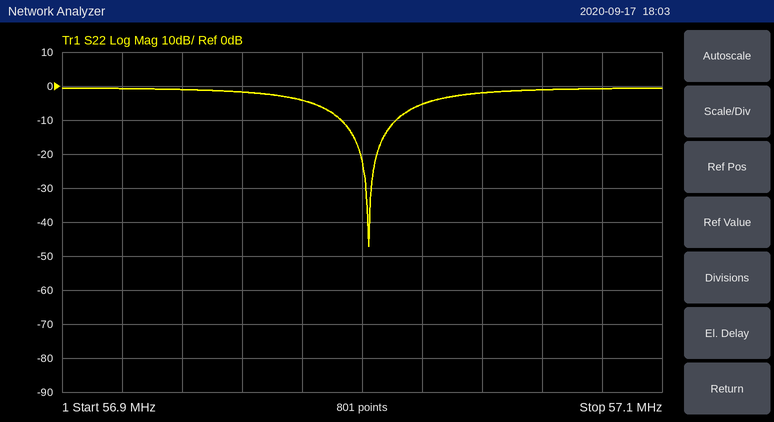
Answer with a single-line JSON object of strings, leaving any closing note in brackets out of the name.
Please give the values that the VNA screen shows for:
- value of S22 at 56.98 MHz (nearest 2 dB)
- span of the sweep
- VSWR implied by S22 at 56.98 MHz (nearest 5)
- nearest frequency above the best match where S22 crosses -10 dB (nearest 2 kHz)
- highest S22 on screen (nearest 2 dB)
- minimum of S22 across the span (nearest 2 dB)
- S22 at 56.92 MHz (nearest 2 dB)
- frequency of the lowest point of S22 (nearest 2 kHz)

{"value of S22 at 56.98 MHz": "-4 dB", "span of the sweep": "200 kHz", "VSWR implied by S22 at 56.98 MHz": "5", "nearest frequency above the best match where S22 crosses -10 dB": "57.012 MHz", "highest S22 on screen": "0 dB", "minimum of S22 across the span": "-48 dB", "S22 at 56.92 MHz": "0 dB", "frequency of the lowest point of S22": "57.002 MHz"}
